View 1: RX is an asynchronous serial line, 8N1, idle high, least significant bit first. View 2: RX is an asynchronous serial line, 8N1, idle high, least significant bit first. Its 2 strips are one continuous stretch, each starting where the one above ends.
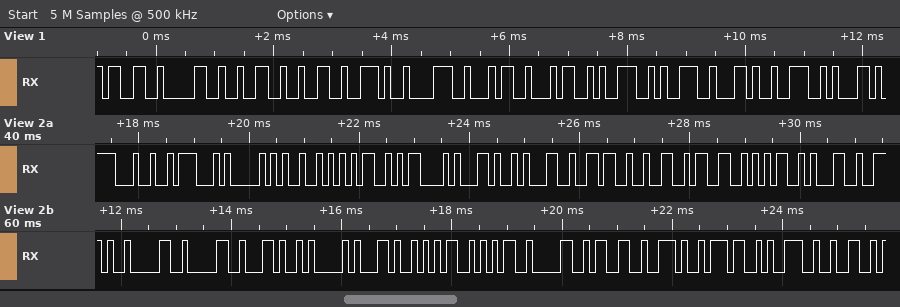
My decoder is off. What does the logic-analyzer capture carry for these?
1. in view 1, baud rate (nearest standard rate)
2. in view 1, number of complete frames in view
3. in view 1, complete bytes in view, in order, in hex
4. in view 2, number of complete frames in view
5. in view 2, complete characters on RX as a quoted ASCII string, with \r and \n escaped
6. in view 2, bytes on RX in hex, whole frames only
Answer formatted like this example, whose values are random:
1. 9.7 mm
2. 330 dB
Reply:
1. 9600 baud
2. 12
3. 0x33 0x30 0x32 0x32 0x2E 0x38 0x34 0x34 0x39 0x39 0x2C 0x4E
4. 27
5. "$GPRMC,162351.00,A,5503.792"
6. 0x24 0x47 0x50 0x52 0x4D 0x43 0x2C 0x31 0x36 0x32 0x33 0x35 0x31 0x2E 0x30 0x30 0x2C 0x41 0x2C 0x35 0x35 0x30 0x33 0x2E 0x37 0x39 0x32
